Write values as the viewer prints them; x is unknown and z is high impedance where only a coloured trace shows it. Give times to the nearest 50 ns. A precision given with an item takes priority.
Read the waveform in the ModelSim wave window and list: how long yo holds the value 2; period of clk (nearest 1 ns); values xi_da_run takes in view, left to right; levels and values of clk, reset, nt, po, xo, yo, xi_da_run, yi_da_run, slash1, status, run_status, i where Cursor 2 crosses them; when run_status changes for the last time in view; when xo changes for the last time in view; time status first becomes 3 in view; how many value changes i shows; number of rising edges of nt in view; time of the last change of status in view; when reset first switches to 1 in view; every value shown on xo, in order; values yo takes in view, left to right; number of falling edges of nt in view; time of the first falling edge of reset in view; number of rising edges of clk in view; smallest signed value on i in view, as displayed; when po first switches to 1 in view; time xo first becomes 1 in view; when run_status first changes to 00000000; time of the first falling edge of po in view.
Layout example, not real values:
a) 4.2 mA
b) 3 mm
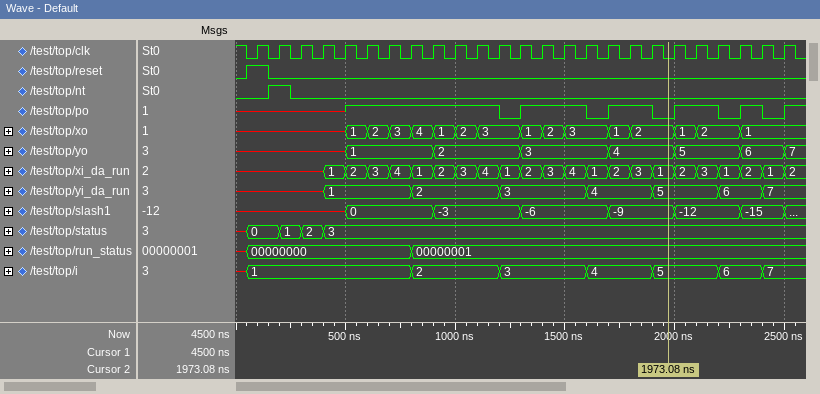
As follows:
a) 400 ns
b) 100 ns
c) x, 1, 2, 3, 4, 1, 2, 3, 4, 1, 2, 3, 4, 1, 2, 3, 1, 2, 3, 1, 2, 1, 2
d) clk=0, reset=0, nt=0, po=0, xo=2, yo=4, xi_da_run=1, yi_da_run=5, slash1=-9, status=3, run_status=00000001, i=5
e) 800 ns
f) 2300 ns
g) 400 ns
h) 7
i) 1
j) 400 ns
k) 50 ns
l) x, 1, 2, 3, 4, 1, 2, 3, 1, 2, 3, 1, 2, 1, 2, 1
m) x, 1, 2, 3, 4, 5, 6, 7
n) 1
o) 150 ns
p) 25
q) 1
r) 500 ns
s) 500 ns
t) 50 ns
u) 1200 ns
